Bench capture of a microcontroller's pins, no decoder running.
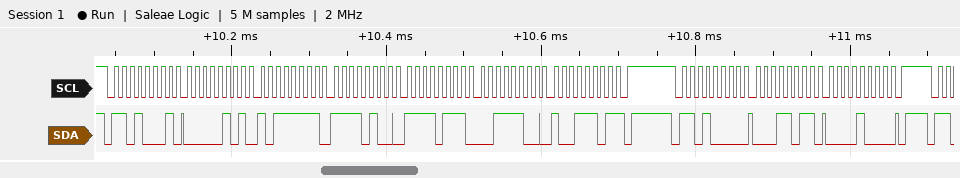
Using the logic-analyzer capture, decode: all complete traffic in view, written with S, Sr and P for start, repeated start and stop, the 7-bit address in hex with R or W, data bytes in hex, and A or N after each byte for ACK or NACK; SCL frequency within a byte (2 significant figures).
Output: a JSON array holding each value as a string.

["S 68R A 05 A BF A F4 A F7 A 3C A 9D N P S 68W A 1B A 08 A P", "100 kHz"]
